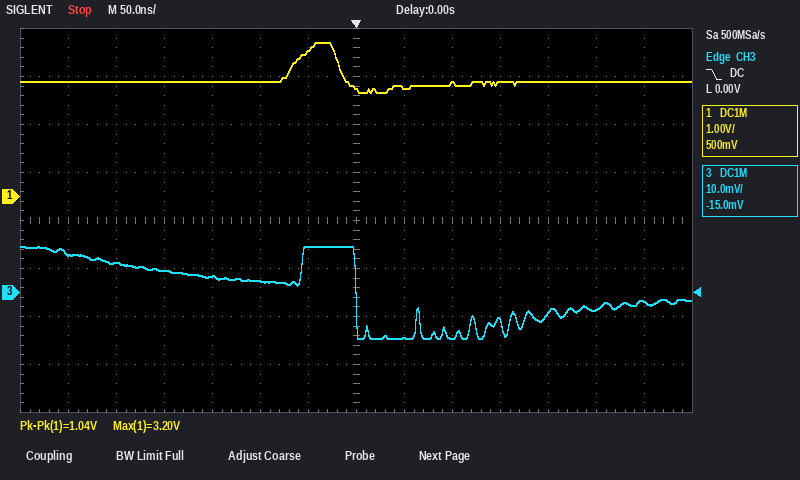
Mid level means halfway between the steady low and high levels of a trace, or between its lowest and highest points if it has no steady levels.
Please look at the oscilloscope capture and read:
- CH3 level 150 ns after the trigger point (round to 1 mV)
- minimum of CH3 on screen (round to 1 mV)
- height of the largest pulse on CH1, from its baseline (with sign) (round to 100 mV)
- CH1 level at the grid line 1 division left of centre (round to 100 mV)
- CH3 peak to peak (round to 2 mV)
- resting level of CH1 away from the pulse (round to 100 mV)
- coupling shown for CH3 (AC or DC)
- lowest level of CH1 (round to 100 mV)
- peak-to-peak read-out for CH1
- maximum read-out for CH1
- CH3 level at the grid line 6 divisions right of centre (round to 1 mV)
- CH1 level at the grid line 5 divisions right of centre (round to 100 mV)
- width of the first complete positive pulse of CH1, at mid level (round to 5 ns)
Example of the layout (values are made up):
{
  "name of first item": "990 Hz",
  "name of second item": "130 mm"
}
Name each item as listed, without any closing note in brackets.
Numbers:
{
  "CH3 level 150 ns after the trigger point": "-6 mV",
  "minimum of CH3 on screen": "-10 mV",
  "height of the largest pulse on CH1, from its baseline (with sign)": "+800 mV",
  "CH1 level at the grid line 1 division left of centre": "3.0 V",
  "CH3 peak to peak": "20 mV",
  "resting level of CH1 away from the pulse": "2.4 V",
  "coupling shown for CH3": "DC",
  "lowest level of CH1": "2.2 V",
  "peak-to-peak read-out for CH1": "1.04 V",
  "maximum read-out for CH1": "3.20 V",
  "CH3 level at the grid line 6 divisions right of centre": "-2 mV",
  "CH1 level at the grid line 5 divisions right of centre": "2.4 V",
  "width of the first complete positive pulse of CH1, at mid level": "50 ns"
}
